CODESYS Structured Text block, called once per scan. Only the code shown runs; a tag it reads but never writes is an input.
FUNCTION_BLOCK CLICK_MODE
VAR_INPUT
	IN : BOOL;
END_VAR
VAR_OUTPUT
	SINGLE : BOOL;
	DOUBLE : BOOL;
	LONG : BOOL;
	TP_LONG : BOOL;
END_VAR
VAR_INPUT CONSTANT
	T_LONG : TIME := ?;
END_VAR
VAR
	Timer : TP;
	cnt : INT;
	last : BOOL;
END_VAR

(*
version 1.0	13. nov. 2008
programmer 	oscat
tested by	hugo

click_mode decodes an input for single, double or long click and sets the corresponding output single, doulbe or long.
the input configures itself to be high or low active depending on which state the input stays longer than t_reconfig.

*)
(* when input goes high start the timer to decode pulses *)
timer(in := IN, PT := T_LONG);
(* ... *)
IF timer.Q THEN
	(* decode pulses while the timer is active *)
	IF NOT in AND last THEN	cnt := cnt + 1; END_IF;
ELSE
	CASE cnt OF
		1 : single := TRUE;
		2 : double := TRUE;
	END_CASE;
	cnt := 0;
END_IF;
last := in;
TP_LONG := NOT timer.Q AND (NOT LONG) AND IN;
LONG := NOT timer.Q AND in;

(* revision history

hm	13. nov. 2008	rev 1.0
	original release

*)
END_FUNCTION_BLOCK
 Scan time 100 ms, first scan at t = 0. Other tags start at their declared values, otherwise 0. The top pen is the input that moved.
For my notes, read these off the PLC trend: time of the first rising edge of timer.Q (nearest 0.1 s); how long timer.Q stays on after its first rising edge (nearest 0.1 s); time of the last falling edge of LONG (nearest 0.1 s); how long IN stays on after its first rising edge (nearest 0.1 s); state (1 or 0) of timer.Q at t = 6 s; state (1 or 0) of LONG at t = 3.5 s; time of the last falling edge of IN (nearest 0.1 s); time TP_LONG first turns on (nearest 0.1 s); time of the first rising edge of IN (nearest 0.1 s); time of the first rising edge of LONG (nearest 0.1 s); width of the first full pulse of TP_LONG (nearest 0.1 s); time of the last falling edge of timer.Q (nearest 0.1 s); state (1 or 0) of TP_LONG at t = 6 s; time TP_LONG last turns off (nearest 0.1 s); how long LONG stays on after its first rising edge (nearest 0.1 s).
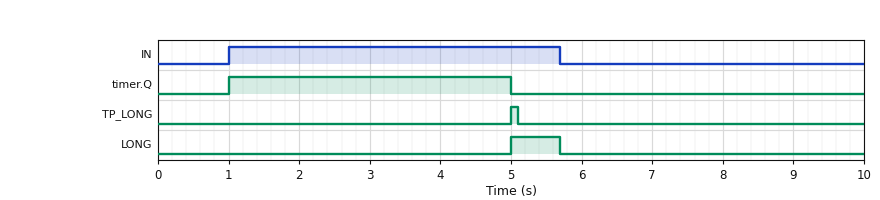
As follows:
1.0 s
4.0 s
5.7 s
4.7 s
0
0
5.7 s
5.0 s
1.0 s
5.0 s
0.1 s
5.0 s
0
5.1 s
0.7 s
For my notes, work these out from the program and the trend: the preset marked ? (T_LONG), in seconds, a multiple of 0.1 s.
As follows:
4.0 s
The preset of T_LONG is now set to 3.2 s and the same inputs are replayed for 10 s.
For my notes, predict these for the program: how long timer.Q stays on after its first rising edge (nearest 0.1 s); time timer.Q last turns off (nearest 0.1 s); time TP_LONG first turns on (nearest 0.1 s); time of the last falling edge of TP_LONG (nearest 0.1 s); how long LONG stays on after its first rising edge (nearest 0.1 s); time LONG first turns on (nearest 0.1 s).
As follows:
3.2 s
4.2 s
4.2 s
4.3 s
1.5 s
4.2 s
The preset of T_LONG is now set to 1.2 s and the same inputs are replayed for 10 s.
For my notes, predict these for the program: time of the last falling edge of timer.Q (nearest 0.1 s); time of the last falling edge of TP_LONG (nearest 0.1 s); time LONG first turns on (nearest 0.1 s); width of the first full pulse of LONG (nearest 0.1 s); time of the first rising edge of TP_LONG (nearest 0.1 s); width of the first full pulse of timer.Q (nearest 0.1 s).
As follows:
2.2 s
2.3 s
2.2 s
3.5 s
2.2 s
1.2 s
